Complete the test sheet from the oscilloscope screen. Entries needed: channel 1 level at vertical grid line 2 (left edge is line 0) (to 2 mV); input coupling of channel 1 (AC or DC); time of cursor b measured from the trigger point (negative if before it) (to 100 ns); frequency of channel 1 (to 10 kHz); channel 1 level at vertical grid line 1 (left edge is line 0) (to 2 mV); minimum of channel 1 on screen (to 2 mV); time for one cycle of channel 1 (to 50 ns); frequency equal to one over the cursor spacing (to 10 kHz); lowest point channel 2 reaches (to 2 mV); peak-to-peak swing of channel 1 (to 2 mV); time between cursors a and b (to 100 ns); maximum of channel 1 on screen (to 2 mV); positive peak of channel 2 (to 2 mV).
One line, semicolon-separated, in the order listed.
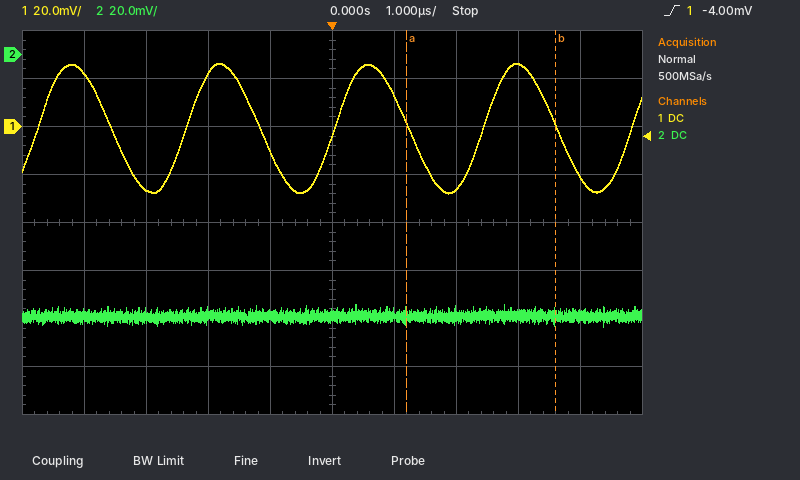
-26 mV; DC; +3.6 µs; 420 kHz; 22 mV; -28 mV; 2.40 µs; 420 kHz; -114 mV; 54 mV; 2.4 µs; 26 mV; -104 mV
